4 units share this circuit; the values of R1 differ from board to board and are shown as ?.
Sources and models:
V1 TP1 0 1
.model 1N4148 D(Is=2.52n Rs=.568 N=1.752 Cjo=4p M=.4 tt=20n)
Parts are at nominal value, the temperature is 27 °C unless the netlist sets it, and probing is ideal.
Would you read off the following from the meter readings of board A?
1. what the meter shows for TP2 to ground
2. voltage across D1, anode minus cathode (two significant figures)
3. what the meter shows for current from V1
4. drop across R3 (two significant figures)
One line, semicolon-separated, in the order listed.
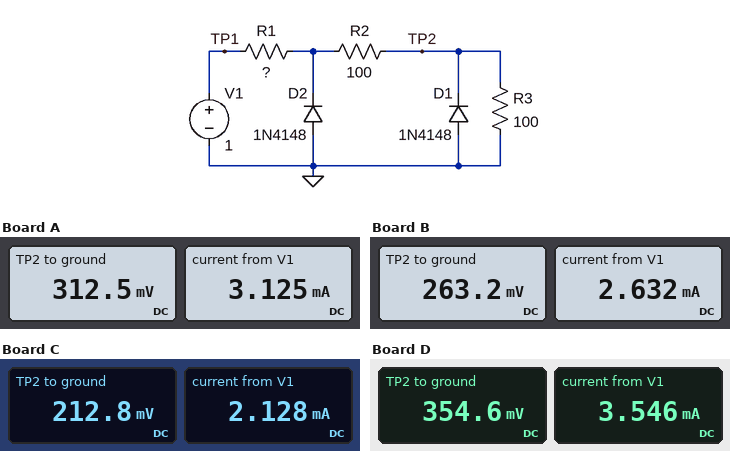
312.5 mV; -310 mV; 3.125 mA; 310 mV
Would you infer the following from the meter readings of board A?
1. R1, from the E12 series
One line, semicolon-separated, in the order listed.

120 Ω
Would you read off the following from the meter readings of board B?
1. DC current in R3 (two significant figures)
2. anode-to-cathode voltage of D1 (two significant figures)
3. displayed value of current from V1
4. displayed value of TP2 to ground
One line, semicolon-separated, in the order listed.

2.6 mA; -260 mV; 2.632 mA; 263.2 mV
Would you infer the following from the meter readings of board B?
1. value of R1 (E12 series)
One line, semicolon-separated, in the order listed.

180 Ω
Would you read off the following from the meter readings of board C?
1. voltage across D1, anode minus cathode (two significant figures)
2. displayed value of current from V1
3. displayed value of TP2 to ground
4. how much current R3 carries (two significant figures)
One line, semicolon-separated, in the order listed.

-210 mV; 2.128 mA; 212.8 mV; 2.1 mA
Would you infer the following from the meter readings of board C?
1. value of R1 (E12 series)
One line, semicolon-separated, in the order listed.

270 Ω
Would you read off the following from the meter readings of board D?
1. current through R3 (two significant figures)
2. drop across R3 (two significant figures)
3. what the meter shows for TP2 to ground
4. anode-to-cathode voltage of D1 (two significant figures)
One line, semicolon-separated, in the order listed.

3.5 mA; 350 mV; 354.6 mV; -350 mV
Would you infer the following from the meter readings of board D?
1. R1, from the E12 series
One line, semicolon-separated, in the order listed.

82 Ω
